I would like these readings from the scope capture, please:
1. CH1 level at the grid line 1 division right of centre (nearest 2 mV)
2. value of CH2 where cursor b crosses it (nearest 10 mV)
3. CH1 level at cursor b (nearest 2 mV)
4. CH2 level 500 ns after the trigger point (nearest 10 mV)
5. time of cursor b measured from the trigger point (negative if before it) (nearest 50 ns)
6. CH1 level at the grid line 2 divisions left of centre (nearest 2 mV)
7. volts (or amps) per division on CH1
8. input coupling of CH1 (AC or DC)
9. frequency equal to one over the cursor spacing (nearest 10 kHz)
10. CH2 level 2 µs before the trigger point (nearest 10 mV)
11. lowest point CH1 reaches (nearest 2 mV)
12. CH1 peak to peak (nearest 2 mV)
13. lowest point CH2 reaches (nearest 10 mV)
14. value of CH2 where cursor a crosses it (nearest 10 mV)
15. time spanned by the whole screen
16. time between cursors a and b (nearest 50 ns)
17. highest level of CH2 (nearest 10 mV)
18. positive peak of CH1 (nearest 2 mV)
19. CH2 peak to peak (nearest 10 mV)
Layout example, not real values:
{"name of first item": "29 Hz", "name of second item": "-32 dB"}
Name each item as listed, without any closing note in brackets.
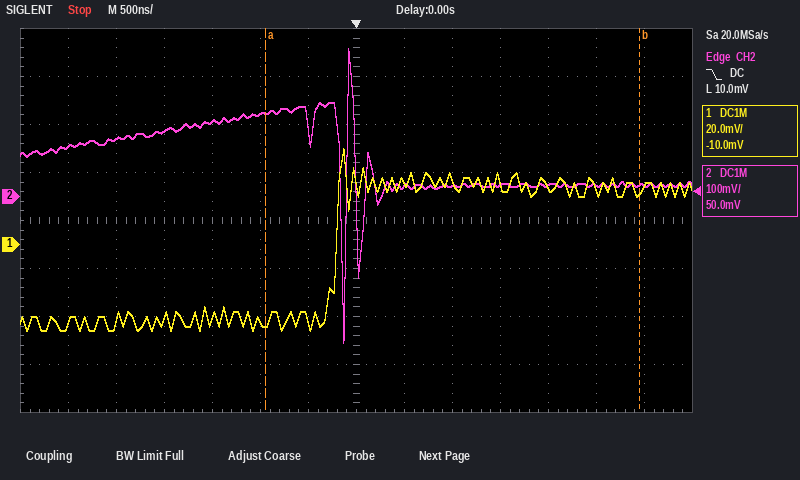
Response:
{"CH1 level at the grid line 1 division right of centre": "26 mV", "value of CH2 where cursor b crosses it": "20 mV", "CH1 level at cursor b": "22 mV", "CH2 level 500 ns after the trigger point": "20 mV", "time of cursor b measured from the trigger point (negative if before it)": "+2.95 µs", "CH1 level at the grid line 2 divisions left of centre": "-32 mV", "volts (or amps) per division on CH1": "20 mV", "input coupling of CH1": "DC", "frequency equal to one over the cursor spacing": "260 kHz", "CH2 level 2 µs before the trigger point": "140 mV", "lowest point CH1 reaches": "-36 mV", "CH1 peak to peak": "76 mV", "lowest point CH2 reaches": "-300 mV", "value of CH2 where cursor a crosses it": "170 mV", "time spanned by the whole screen": "7 µs", "time between cursors a and b": "3.90 µs", "highest level of CH2": "310 mV", "positive peak of CH1": "40 mV", "CH2 peak to peak": "610 mV"}
